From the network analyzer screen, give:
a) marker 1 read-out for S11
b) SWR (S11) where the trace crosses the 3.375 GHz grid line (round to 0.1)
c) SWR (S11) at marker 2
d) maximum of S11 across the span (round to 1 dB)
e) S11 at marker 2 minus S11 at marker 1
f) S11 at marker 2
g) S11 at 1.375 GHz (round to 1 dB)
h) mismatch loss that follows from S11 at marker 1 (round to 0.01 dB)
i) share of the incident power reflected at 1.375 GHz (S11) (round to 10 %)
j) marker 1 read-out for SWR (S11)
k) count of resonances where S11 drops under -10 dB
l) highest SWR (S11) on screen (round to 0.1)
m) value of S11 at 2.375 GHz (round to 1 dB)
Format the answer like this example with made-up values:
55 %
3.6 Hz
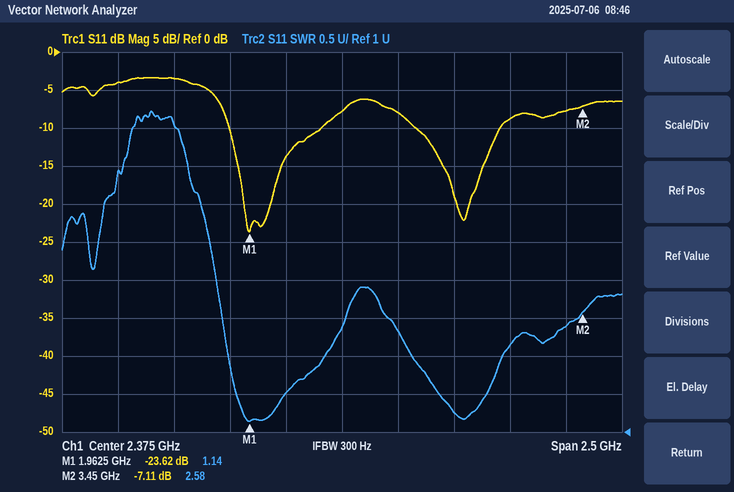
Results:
-23.62 dB
2.4
2.58
-3 dB
16.51 dB
-7.11 dB
-4 dB
0.02 dB
40 %
1.14
2
5.2
-8 dB
